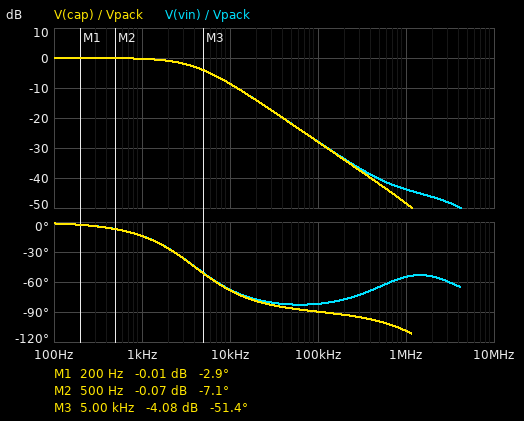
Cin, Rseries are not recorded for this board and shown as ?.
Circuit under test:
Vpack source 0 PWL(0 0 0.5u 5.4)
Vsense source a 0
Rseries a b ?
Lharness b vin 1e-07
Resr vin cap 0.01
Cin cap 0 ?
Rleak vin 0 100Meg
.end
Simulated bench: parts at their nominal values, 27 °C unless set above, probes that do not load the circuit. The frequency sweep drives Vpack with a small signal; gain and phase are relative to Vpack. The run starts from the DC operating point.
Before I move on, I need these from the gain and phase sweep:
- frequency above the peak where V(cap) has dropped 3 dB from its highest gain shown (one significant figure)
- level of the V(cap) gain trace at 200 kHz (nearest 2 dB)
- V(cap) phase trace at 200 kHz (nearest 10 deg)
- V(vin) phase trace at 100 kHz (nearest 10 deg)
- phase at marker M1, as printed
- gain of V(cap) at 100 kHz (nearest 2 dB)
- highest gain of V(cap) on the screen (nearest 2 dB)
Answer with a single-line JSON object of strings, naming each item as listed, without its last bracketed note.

{"frequency above the peak where V(cap) has dropped 3 dB from its highest gain shown": "4 kHz", "level of the V(cap) gain trace at 200 kHz": "-34 dB", "V(cap) phase trace at 200 kHz": "-90 deg", "V(vin) phase trace at 100 kHz": "-80 deg", "phase at marker M1, as printed": "-2.9 deg", "gain of V(cap) at 100 kHz": "-28 dB", "highest gain of V(cap) on the screen": "0 dB"}
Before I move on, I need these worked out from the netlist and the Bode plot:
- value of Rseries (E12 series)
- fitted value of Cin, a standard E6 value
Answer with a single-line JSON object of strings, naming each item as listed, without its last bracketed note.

{"value of Rseries": "1.8 Ω", "fitted value of Cin, a standard E6 value": "22 µF"}
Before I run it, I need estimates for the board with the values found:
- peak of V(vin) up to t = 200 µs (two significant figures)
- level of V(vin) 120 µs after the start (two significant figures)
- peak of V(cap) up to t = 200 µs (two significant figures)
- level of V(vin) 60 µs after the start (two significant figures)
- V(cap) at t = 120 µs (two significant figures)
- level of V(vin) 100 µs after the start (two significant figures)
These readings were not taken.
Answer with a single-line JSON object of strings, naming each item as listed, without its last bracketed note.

{"peak of V(vin) up to t = 200 µs": "5.4 V", "level of V(vin) 120 µs after the start": "5.1 V", "peak of V(cap) up to t = 200 µs": "5.4 V", "level of V(vin) 60 µs after the start": "4.2 V", "V(cap) at t = 120 µs": "5.1 V", "level of V(vin) 100 µs after the start": "5.0 V"}
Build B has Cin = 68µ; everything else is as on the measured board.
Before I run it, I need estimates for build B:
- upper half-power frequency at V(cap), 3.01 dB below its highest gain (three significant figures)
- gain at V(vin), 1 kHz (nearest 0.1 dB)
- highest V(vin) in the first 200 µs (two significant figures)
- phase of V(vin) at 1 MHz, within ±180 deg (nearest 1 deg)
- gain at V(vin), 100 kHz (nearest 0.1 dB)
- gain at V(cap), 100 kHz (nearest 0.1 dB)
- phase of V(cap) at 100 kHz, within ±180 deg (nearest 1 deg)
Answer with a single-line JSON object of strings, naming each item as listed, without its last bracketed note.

{"upper half-power frequency at V(cap), 3.01 dB below its highest gain": "1.29 kHz", "gain at V(vin), 1 kHz": "-2.0 dB", "highest V(vin) in the first 200 µs": "4.3 V", "phase of V(vin) at 1 MHz, within ±180 deg": "-32 deg", "gain at V(vin), 100 kHz": "-37.0 dB", "gain at V(cap), 100 kHz": "-37.8 dB", "phase of V(cap) at 100 kHz, within ±180 deg": "-91 deg"}
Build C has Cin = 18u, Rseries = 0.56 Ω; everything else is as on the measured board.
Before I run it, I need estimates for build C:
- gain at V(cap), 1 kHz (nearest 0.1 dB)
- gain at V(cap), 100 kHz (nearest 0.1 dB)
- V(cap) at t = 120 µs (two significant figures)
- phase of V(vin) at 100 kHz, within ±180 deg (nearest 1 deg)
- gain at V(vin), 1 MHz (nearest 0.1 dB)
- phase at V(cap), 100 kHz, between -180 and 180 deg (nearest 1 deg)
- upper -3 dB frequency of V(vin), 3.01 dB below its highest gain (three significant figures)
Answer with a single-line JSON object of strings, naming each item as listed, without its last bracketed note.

{"gain at V(cap), 1 kHz": "0 dB", "gain at V(cap), 100 kHz": "-16.2 dB", "V(cap) at t = 120 µs": "5.4 V", "phase of V(vin) at 100 kHz, within ±180 deg": "-81 deg", "gain at V(vin), 1 MHz": "-36.0 dB", "phase at V(cap), 100 kHz, between -180 and 180 deg": "-87 deg", "upper -3 dB frequency of V(vin), 3.01 dB below its highest gain": "15.8 kHz"}
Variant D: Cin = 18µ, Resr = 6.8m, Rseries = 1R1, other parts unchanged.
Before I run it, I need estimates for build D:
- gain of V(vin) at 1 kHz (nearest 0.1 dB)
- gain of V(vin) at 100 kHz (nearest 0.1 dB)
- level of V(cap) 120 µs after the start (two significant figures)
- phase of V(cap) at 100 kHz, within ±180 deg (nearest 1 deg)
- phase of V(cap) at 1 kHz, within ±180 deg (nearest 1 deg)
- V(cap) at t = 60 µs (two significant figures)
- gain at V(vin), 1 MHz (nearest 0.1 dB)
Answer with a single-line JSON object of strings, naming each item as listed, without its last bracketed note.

{"gain of V(vin) at 1 kHz": "-0.1 dB", "gain of V(vin) at 100 kHz": "-21.9 dB", "level of V(cap) 120 µs after the start": "5.4 V", "phase of V(cap) at 100 kHz, within ±180 deg": "-89 deg", "phase of V(cap) at 1 kHz, within ±180 deg": "-7 deg", "V(cap) at t = 60 µs": "5.1 V", "gain at V(vin), 1 MHz": "-41.1 dB"}
